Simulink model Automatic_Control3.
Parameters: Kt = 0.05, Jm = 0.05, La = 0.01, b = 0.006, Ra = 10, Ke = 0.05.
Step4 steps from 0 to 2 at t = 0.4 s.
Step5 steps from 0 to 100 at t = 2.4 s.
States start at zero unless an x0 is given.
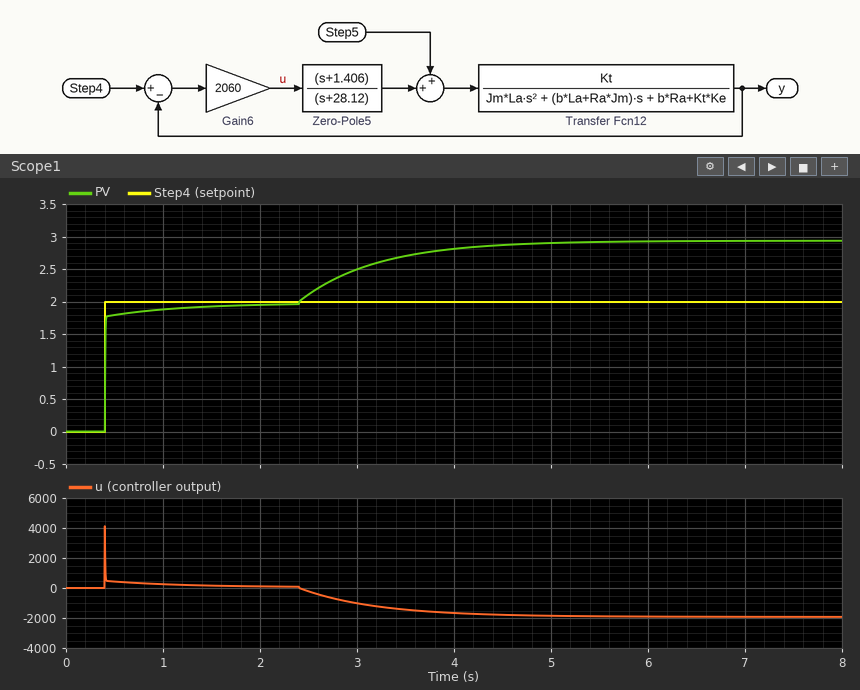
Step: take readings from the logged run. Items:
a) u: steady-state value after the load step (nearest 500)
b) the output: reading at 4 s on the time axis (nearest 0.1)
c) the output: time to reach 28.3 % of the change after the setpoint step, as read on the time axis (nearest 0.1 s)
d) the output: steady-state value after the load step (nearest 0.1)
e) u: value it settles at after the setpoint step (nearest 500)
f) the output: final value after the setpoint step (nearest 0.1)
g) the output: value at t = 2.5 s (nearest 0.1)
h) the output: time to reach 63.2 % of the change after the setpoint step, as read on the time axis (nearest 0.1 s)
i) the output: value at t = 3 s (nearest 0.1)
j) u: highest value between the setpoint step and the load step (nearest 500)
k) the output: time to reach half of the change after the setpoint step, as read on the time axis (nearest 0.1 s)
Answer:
-2000
2.8
0.4 s
2.9
0
2.0
2.1
0.4 s
2.5
4000
0.4 s
